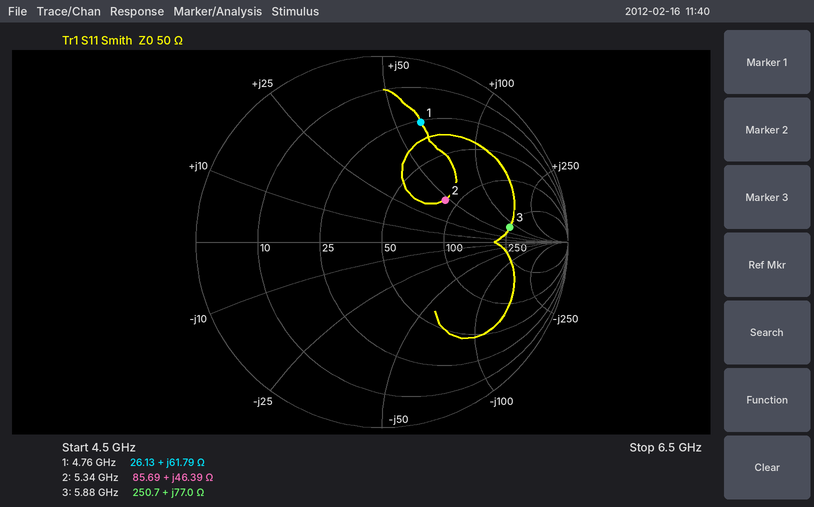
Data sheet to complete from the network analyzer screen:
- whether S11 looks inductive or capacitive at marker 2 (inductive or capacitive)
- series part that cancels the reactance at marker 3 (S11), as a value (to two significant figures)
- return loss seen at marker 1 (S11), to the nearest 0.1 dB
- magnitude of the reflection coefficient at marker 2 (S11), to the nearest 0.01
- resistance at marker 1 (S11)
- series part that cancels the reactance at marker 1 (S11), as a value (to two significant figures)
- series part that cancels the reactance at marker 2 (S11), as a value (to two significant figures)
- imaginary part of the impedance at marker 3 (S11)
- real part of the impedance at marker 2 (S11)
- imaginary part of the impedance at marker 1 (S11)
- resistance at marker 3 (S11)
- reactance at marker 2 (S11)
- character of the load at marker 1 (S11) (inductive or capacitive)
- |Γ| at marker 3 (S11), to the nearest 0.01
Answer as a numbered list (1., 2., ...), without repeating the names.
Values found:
1. inductive
2. 350 fF
3. 3.4 dB
4. 0.41
5. 26.13 Ω
6. 540 fF
7. 640 fF
8. +77.0 Ω
9. 85.69 Ω
10. +61.79 Ω
11. 250.7 Ω
12. +46.39 Ω
13. inductive
14. 0.69
